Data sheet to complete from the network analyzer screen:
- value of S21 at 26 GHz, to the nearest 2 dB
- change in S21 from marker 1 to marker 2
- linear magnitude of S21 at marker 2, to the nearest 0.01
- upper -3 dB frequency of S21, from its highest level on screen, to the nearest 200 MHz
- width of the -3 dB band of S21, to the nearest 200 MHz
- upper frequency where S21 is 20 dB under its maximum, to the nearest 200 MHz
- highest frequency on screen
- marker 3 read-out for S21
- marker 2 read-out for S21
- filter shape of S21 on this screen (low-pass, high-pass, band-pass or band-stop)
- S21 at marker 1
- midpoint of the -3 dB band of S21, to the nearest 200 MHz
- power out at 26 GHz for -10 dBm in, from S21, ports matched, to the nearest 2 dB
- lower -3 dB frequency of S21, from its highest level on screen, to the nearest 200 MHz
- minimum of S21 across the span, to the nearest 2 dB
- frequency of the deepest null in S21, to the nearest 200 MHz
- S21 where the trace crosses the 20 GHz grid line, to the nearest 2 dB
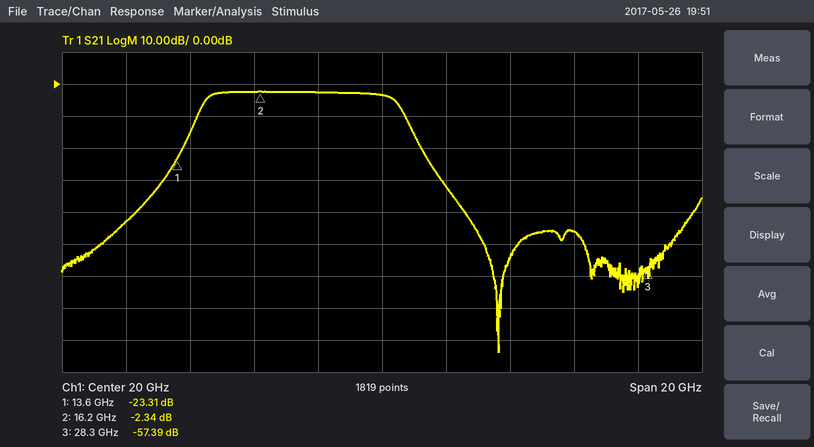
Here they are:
-46 dB
20.97 dB
0.76
20.4 GHz
6.0 GHz
21.4 GHz
30 GHz
-57.39 dB
-2.34 dB
band-pass
-23.31 dB
17.4 GHz
-56 dBm
14.4 GHz
-84 dB
23.6 GHz
-4 dB
